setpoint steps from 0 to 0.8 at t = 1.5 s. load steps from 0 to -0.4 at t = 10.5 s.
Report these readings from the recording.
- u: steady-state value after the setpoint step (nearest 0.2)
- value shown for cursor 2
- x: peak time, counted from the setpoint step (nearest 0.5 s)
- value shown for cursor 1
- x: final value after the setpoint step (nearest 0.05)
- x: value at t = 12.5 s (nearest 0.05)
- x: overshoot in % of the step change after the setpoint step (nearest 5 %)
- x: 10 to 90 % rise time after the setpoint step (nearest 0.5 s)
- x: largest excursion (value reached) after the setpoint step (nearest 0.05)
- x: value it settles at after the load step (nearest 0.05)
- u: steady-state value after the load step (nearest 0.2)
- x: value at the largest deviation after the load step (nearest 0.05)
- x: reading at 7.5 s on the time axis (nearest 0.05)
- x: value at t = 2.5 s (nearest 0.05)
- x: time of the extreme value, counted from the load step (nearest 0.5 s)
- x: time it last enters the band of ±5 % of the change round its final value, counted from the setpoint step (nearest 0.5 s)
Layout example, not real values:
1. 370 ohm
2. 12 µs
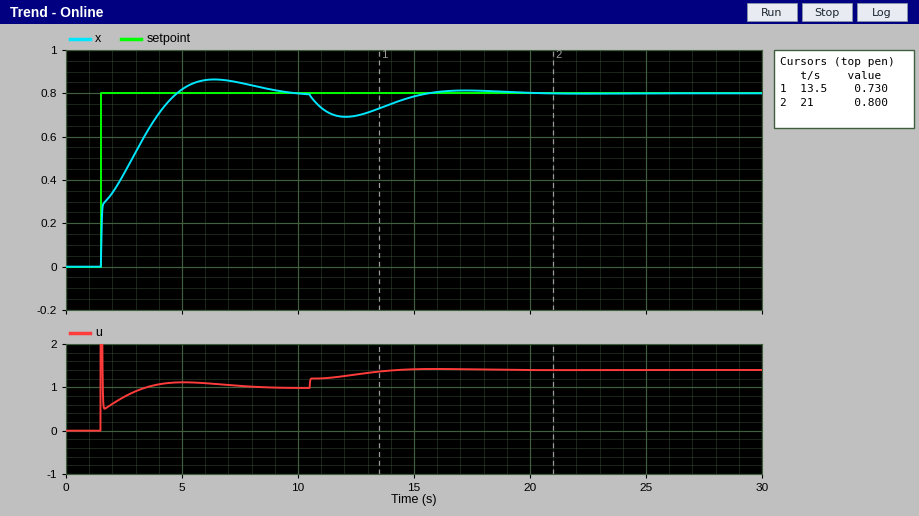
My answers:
1. 1.0
2. 0.800
3. 5.0 s
4. 0.730
5. 0.80
6. 0.70
7. 10 %
8. 2.5 s
9. 0.85
10. 0.80
11. 1.4
12. 0.70
13. 0.85
14. 0.45
15. 1.5 s
16. 6.5 s
